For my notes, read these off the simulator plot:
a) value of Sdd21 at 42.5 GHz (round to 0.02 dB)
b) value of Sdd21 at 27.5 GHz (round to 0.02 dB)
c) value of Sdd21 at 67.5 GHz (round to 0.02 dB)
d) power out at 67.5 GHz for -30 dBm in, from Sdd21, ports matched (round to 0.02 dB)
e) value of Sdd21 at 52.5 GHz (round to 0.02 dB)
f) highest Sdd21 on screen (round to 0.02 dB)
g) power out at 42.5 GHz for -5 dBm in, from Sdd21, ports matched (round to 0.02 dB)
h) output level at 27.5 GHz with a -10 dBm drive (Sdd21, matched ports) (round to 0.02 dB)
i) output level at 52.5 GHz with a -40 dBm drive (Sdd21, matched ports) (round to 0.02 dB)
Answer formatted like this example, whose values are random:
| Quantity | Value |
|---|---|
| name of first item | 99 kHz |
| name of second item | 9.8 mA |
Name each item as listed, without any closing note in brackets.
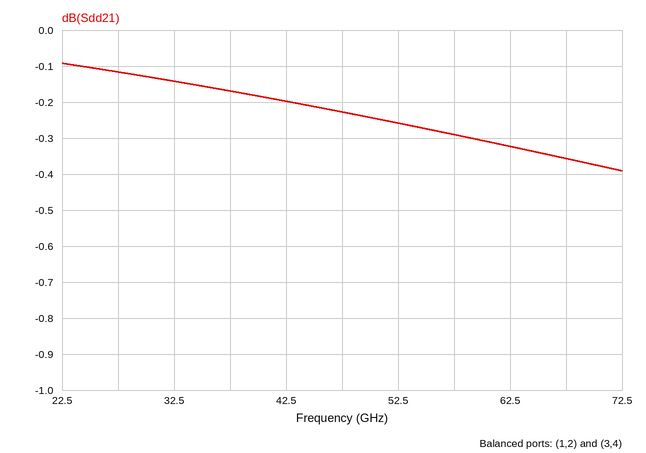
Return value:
| Quantity | Value |
|---|---|
| value of Sdd21 at 42.5 GHz | -0.20 dB |
| value of Sdd21 at 27.5 GHz | -0.12 dB |
| value of Sdd21 at 67.5 GHz | -0.36 dB |
| power out at 67.5 GHz for -30 dBm in, from Sdd21, ports matched | -30.36 dBm |
| value of Sdd21 at 52.5 GHz | -0.26 dB |
| highest Sdd21 on screen | -0.10 dB |
| power out at 42.5 GHz for -5 dBm in, from Sdd21, ports matched | -5.20 dBm |
| output level at 27.5 GHz with a -10 dBm drive (Sdd21, matched ports) | -10.12 dBm |
| output level at 52.5 GHz with a -40 dBm drive (Sdd21, matched ports) | -40.26 dBm |
